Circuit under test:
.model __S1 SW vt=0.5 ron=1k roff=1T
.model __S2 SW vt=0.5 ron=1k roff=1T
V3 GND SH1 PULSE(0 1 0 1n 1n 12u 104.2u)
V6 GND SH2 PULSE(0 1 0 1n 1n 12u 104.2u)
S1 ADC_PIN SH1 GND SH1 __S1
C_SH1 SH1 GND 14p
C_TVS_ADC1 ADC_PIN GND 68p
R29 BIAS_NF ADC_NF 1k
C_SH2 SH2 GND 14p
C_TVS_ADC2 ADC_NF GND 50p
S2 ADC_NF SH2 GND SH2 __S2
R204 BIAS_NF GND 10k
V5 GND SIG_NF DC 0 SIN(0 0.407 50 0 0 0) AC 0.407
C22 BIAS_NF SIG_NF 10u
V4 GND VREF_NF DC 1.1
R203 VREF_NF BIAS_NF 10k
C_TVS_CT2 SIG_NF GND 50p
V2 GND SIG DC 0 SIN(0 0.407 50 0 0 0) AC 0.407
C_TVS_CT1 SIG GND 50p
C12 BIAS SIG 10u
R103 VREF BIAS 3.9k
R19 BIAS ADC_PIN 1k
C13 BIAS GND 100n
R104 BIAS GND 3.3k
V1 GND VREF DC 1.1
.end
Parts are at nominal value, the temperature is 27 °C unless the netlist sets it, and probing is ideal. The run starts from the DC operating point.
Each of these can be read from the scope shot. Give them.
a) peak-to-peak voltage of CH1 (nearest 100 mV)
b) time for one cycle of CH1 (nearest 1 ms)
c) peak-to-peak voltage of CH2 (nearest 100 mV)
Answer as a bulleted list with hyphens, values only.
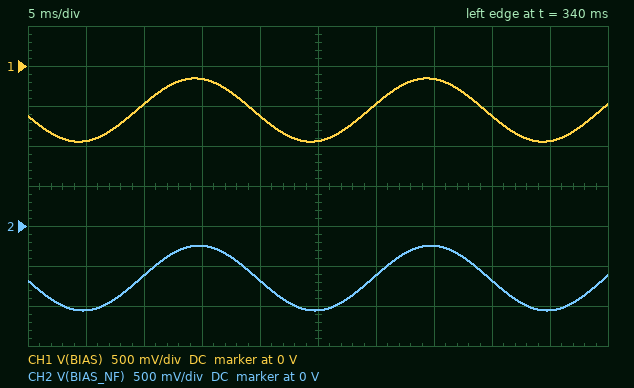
- 800 mV
- 20 ms
- 800 mV
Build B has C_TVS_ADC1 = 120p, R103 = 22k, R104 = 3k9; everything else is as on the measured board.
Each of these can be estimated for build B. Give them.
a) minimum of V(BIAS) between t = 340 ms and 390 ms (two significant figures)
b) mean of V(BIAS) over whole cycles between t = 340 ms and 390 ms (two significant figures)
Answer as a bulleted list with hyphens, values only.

- -700 mV
- -300 mV
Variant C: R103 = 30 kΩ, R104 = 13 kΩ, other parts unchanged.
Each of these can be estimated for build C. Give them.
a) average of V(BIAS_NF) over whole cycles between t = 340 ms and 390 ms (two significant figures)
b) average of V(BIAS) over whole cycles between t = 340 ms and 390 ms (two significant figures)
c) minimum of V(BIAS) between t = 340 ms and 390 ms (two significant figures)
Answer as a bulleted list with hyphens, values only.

- -650 mV
- -560 mV
- -960 mV
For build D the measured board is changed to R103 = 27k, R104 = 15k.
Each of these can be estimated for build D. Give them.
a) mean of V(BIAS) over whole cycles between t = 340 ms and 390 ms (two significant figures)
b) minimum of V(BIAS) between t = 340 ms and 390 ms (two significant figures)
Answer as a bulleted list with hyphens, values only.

- -610 mV
- -1.0 V
